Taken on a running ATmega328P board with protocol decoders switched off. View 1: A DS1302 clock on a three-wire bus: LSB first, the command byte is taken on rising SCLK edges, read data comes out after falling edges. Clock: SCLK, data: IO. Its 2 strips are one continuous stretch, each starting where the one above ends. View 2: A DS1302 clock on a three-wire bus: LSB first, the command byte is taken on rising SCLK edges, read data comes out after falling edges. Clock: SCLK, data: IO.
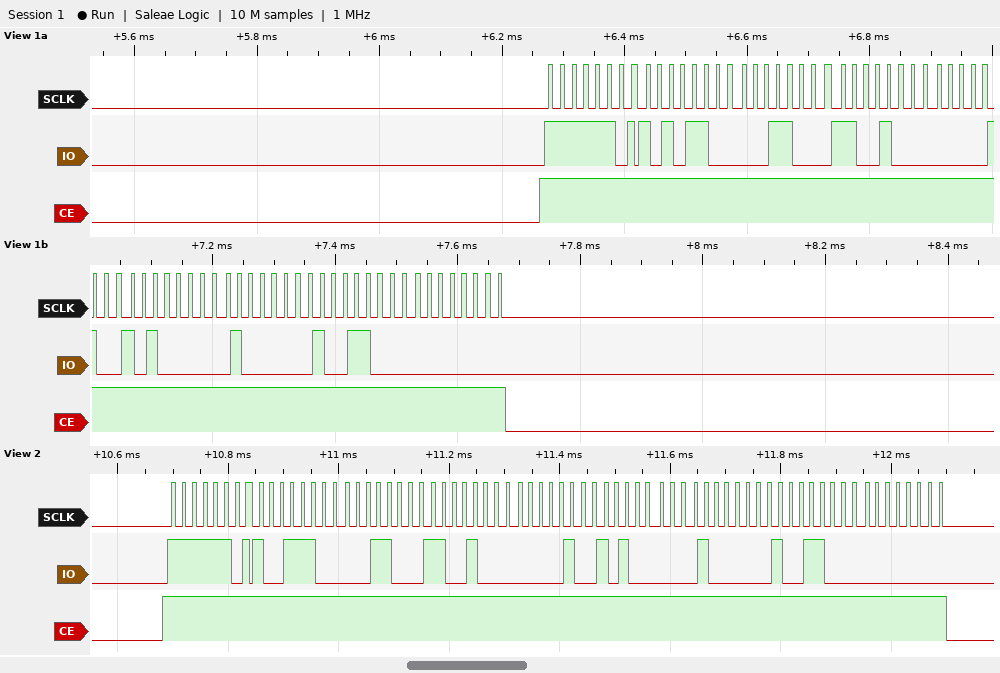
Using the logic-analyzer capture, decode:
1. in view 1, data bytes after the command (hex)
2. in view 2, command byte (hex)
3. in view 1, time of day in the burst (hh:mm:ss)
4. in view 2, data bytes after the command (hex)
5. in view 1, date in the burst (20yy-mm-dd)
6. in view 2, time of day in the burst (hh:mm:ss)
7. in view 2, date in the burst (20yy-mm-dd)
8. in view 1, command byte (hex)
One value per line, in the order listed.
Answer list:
35 18 13 20 05 02 19 00
0xBF
13:18:35
39 18 13 20 05 02 19 00
2019-05-20
13:18:39
2019-05-20
0xBF
